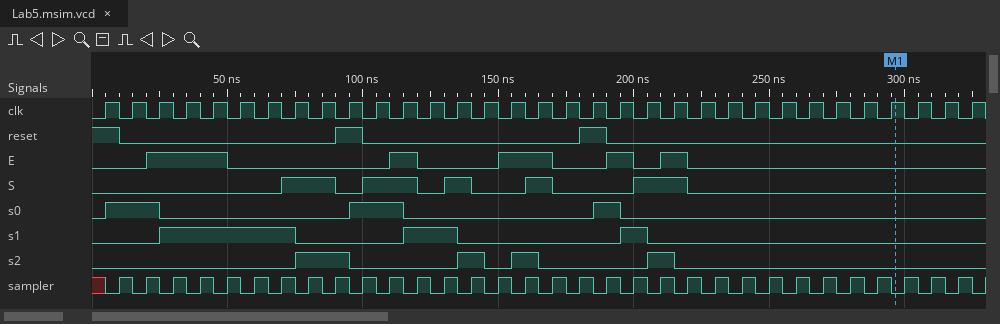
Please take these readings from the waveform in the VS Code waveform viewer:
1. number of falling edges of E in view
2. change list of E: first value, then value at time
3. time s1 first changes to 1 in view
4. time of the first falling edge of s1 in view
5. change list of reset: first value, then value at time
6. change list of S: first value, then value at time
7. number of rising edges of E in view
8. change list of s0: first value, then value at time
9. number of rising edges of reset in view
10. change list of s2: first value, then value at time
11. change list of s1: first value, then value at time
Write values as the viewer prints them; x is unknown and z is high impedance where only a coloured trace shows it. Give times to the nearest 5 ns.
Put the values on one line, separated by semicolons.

5; 0, 1 at 20 ns, 0 at 50 ns, 1 at 110 ns, 0 at 120 ns, 1 at 150 ns, 0 at 170 ns, 1 at 190 ns, 0 at 200 ns, 1 at 210 ns, 0 at 220 ns; 25 ns; 75 ns; 1, 0 at 10 ns, 1 at 90 ns, 0 at 100 ns, 1 at 180 ns, 0 at 190 ns; 0, 1 at 70 ns, 0 at 90 ns, 1 at 100 ns, 0 at 120 ns, 1 at 130 ns, 0 at 140 ns, 1 at 160 ns, 0 at 170 ns, 1 at 200 ns, 0 at 220 ns; 5; 0, 1 at 5 ns, 0 at 25 ns, 1 at 95 ns, 0 at 115 ns, 1 at 185 ns, 0 at 195 ns; 2; 0, 1 at 75 ns, 0 at 95 ns, 1 at 135 ns, 0 at 145 ns, 1 at 155 ns, 0 at 165 ns, 1 at 205 ns, 0 at 215 ns; 0, 1 at 25 ns, 0 at 75 ns, 1 at 115 ns, 0 at 135 ns, 1 at 195 ns, 0 at 205 ns
